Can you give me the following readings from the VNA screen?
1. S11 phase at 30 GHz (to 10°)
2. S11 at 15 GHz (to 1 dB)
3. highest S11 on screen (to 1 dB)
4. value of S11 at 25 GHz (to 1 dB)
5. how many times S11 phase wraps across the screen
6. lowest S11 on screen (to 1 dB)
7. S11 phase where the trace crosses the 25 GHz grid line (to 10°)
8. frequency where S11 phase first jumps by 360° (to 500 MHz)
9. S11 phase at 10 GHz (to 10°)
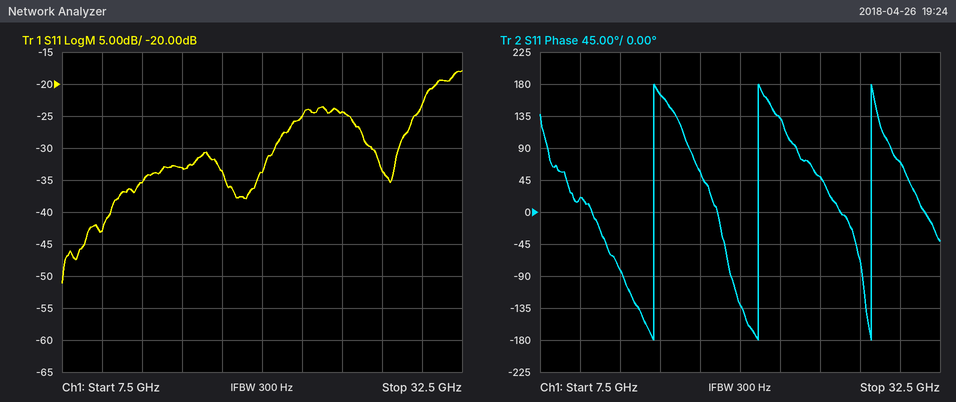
70°
-33 dB
-18 dB
-24 dB
3
-51 dB
50°
14.5 GHz
20°
